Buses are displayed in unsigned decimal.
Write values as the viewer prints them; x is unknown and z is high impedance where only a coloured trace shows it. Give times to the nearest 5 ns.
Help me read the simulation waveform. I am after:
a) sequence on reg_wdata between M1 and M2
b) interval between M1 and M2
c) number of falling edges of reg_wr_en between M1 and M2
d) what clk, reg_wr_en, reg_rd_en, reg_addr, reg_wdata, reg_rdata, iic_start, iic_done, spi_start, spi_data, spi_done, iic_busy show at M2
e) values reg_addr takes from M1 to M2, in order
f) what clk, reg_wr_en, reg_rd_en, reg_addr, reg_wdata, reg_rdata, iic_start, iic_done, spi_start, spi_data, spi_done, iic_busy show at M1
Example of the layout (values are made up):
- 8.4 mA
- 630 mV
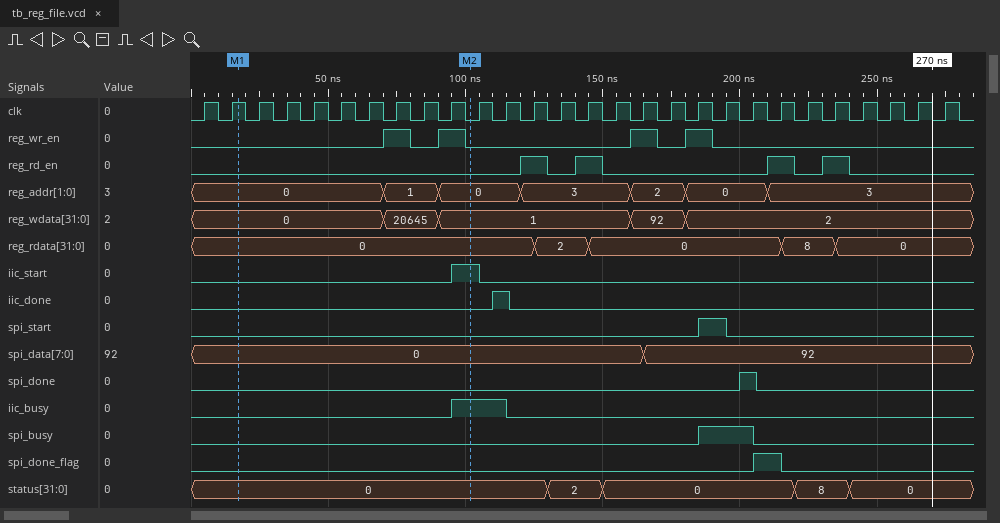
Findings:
- 0, 20645, 1
- 85 ns
- 2
- clk=0, reg_wr_en=0, reg_rd_en=0, reg_addr=0, reg_wdata=1, reg_rdata=0, iic_start=1, iic_done=0, spi_start=0, spi_data=0, spi_done=0, iic_busy=1
- 0, 1, 0
- clk=1, reg_wr_en=0, reg_rd_en=0, reg_addr=0, reg_wdata=0, reg_rdata=0, iic_start=0, iic_done=0, spi_start=0, spi_data=0, spi_done=0, iic_busy=0
